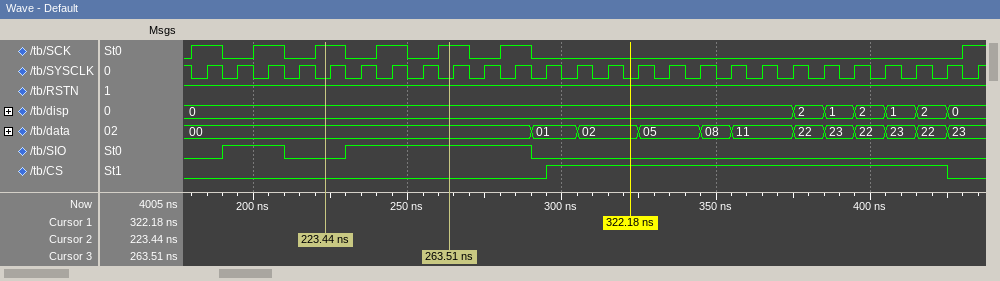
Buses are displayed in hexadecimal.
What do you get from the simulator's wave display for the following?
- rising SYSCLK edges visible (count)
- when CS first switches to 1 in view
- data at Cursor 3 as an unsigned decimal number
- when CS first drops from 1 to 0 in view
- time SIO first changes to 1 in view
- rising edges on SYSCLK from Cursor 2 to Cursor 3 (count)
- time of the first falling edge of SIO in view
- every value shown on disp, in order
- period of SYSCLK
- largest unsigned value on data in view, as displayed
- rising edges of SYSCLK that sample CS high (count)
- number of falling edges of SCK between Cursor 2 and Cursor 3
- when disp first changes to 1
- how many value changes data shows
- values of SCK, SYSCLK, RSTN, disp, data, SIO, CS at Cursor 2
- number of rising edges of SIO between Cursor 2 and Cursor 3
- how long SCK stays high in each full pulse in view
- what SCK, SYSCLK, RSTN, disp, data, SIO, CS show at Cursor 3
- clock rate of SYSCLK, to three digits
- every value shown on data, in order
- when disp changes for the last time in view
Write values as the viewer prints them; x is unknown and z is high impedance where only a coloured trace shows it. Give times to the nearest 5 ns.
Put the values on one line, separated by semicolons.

26; 295 ns; 0; 425 ns; 190 ns; 4; 210 ns; 0, 2, 1, 2, 1, 2, 0; 10 ns; 23; 13; 2; 385 ns; 11; SCK=1, SYSCLK=0, RSTN=1, disp=0, data=00, SIO=0, CS=0; 1; 10 ns, 10 ns, 10 ns, 10 ns, 10 ns, 10 ns; SCK=1, SYSCLK=0, RSTN=1, disp=0, data=00, SIO=1, CS=0; 100 MHz; 00, 01, 02, 05, 08, 11, 22, 23, 22, 23, 22, 23; 425 ns
